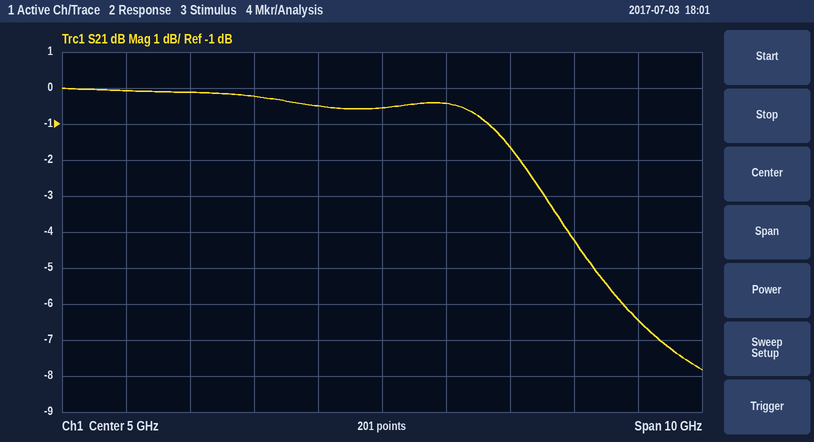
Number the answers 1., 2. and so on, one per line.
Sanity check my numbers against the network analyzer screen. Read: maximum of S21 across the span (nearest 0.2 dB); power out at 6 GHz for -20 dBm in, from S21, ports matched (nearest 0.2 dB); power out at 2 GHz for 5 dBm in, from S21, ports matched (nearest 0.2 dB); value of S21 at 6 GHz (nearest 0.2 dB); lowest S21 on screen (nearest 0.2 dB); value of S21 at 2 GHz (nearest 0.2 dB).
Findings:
1. 0.0 dB
2. -20.4 dBm
3. 4.8 dBm
4. -0.4 dB
5. -7.8 dB
6. -0.2 dB
